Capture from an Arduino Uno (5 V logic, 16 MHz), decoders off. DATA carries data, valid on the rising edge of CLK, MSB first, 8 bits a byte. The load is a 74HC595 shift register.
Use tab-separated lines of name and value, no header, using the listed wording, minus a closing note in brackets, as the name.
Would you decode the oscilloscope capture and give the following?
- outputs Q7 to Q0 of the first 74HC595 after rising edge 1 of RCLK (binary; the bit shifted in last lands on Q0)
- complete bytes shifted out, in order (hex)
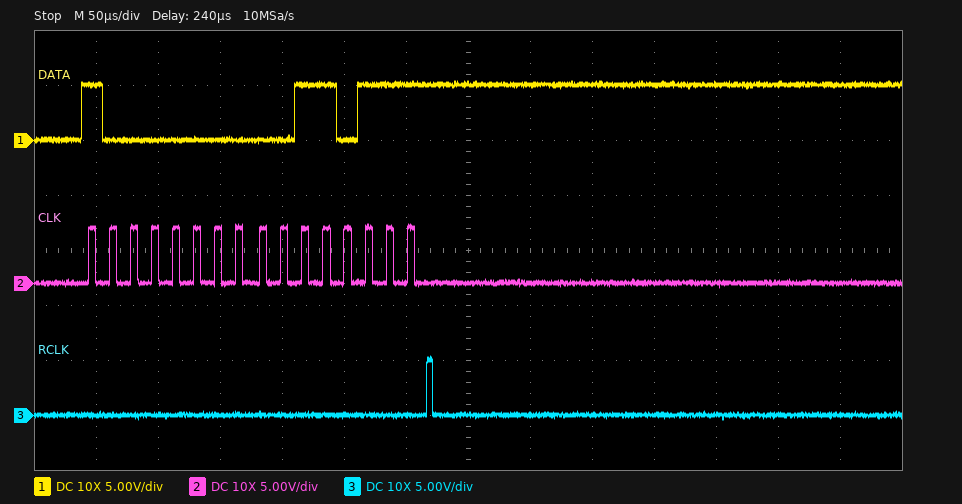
outputs Q7 to Q0 of the first 74HC595 after rising edge 1 of RCLK	00110111
complete bytes shifted out, in order	80 37
